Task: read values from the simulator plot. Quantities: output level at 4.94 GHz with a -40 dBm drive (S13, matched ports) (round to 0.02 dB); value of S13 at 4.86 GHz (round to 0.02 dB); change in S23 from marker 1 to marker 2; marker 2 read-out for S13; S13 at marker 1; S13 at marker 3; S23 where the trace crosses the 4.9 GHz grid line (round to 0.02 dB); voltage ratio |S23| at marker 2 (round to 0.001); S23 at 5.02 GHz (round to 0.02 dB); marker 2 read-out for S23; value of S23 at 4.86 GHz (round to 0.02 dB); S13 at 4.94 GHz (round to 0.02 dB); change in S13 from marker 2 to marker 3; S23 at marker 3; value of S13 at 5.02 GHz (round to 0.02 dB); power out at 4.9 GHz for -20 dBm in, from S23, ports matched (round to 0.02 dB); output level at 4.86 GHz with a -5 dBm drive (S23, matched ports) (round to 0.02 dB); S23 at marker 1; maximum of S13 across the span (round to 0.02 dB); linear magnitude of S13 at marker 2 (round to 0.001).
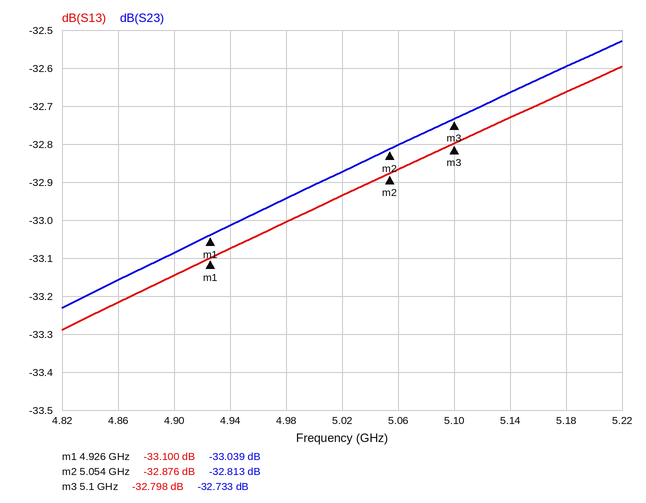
-73.08 dBm
-33.22 dB
0.226 dB
-32.876 dB
-33.100 dB
-32.798 dB
-33.08 dB
0.023
-32.88 dB
-32.813 dB
-33.16 dB
-33.08 dB
0.078 dB
-32.733 dB
-32.94 dB
-53.08 dBm
-38.16 dBm
-33.039 dB
-32.60 dB
0.023
